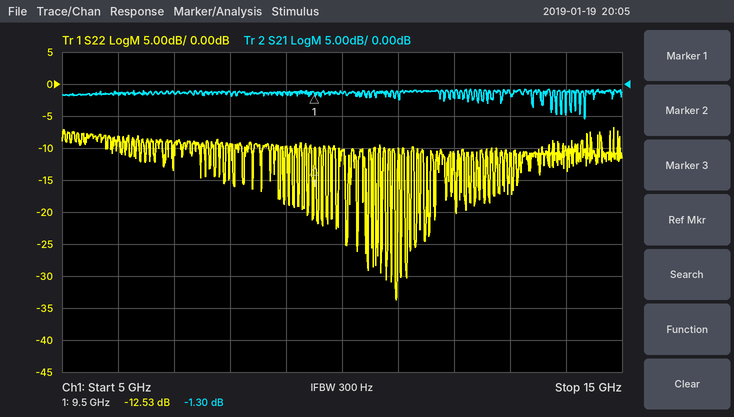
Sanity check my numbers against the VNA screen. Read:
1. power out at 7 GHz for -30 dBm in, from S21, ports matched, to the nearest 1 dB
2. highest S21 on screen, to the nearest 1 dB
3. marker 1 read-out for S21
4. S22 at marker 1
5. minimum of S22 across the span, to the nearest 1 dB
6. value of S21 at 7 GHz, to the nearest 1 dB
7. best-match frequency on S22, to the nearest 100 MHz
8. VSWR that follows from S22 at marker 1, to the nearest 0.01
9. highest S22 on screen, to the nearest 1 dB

-31 dBm
-1 dB
-1.30 dB
-12.53 dB
-34 dB
-1 dB
11.0 GHz
1.62
-7 dB
